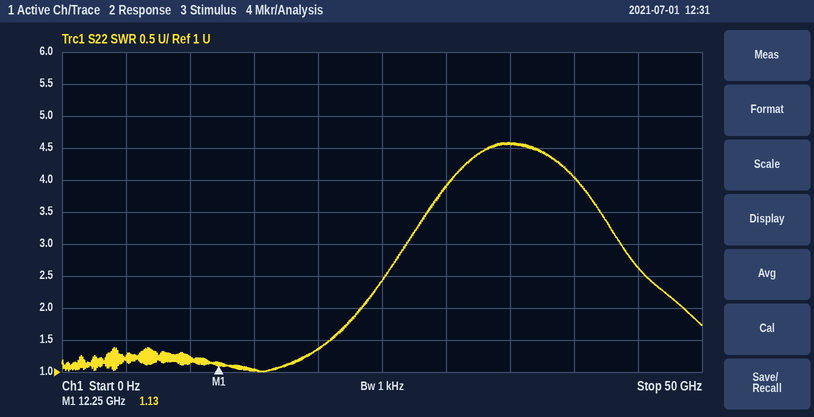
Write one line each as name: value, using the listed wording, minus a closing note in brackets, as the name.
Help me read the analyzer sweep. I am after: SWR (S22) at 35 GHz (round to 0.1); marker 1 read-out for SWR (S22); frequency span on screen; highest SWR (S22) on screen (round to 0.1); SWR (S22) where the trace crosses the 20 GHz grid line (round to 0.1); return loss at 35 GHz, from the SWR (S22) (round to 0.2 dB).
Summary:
SWR (S22) at 35 GHz: 4.6
marker 1 read-out for SWR: 1.13
frequency span on screen: 50 GHz
highest SWR (S22) on screen: 4.6
SWR (S22) where the trace crosses the 20 GHz grid line: 1.4
return loss at 35 GHz, from the SWR (S22): 3.8 dB
